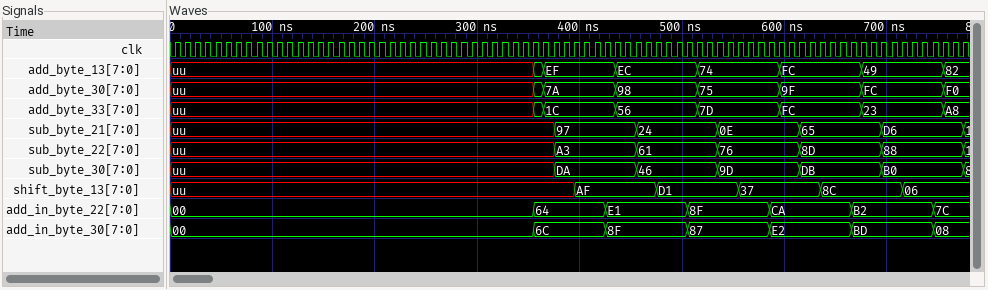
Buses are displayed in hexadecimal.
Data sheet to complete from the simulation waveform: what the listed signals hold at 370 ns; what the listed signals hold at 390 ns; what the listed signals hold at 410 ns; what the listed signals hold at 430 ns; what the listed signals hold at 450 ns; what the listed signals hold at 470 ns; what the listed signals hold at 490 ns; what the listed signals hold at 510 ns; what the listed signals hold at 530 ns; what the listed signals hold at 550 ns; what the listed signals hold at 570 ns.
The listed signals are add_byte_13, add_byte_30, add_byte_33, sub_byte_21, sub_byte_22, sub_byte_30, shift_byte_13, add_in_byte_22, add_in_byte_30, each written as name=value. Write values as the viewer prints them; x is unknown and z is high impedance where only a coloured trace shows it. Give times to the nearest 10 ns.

add_byte_13=EF, add_byte_30=7A, add_byte_33=1C, sub_byte_21=uu, sub_byte_22=uu, sub_byte_30=uu, shift_byte_13=uu, add_in_byte_22=64, add_in_byte_30=6C
add_byte_13=EF, add_byte_30=7A, add_byte_33=1C, sub_byte_21=97, sub_byte_22=A3, sub_byte_30=DA, shift_byte_13=uu, add_in_byte_22=64, add_in_byte_30=6C
add_byte_13=EF, add_byte_30=7A, add_byte_33=1C, sub_byte_21=97, sub_byte_22=A3, sub_byte_30=DA, shift_byte_13=AF, add_in_byte_22=64, add_in_byte_30=6C
add_byte_13=EF, add_byte_30=7A, add_byte_33=1C, sub_byte_21=97, sub_byte_22=A3, sub_byte_30=DA, shift_byte_13=AF, add_in_byte_22=E1, add_in_byte_30=8F
add_byte_13=EC, add_byte_30=98, add_byte_33=56, sub_byte_21=97, sub_byte_22=A3, sub_byte_30=DA, shift_byte_13=AF, add_in_byte_22=E1, add_in_byte_30=8F
add_byte_13=EC, add_byte_30=98, add_byte_33=56, sub_byte_21=24, sub_byte_22=61, sub_byte_30=46, shift_byte_13=AF, add_in_byte_22=E1, add_in_byte_30=8F
add_byte_13=EC, add_byte_30=98, add_byte_33=56, sub_byte_21=24, sub_byte_22=61, sub_byte_30=46, shift_byte_13=D1, add_in_byte_22=E1, add_in_byte_30=8F
add_byte_13=EC, add_byte_30=98, add_byte_33=56, sub_byte_21=24, sub_byte_22=61, sub_byte_30=46, shift_byte_13=D1, add_in_byte_22=8F, add_in_byte_30=87
add_byte_13=74, add_byte_30=75, add_byte_33=7D, sub_byte_21=24, sub_byte_22=61, sub_byte_30=46, shift_byte_13=D1, add_in_byte_22=8F, add_in_byte_30=87
add_byte_13=74, add_byte_30=75, add_byte_33=7D, sub_byte_21=0E, sub_byte_22=76, sub_byte_30=9D, shift_byte_13=D1, add_in_byte_22=8F, add_in_byte_30=87
add_byte_13=74, add_byte_30=75, add_byte_33=7D, sub_byte_21=0E, sub_byte_22=76, sub_byte_30=9D, shift_byte_13=37, add_in_byte_22=8F, add_in_byte_30=87
